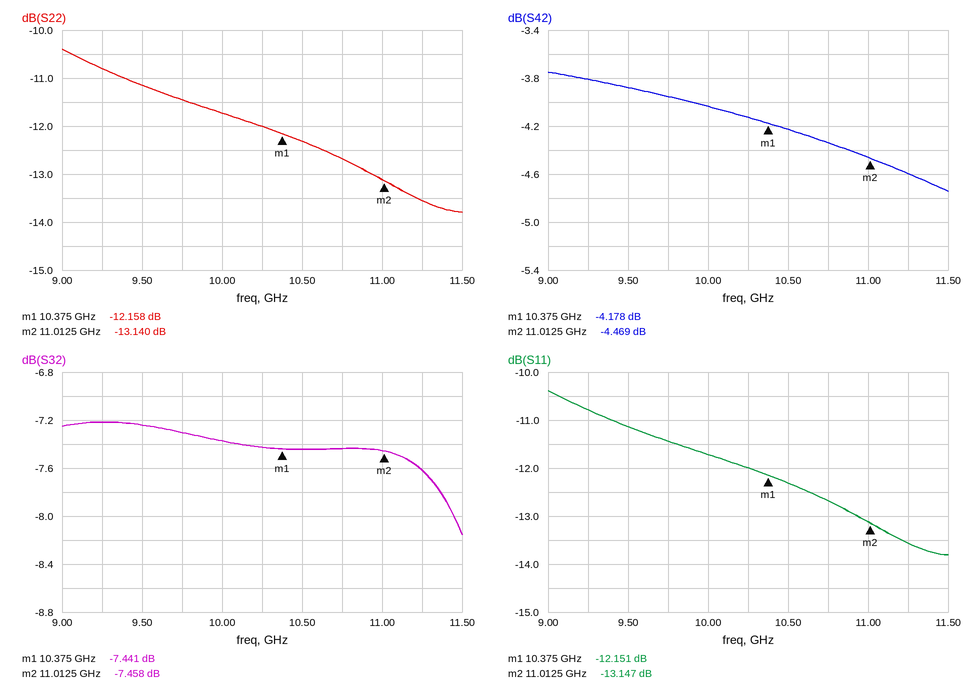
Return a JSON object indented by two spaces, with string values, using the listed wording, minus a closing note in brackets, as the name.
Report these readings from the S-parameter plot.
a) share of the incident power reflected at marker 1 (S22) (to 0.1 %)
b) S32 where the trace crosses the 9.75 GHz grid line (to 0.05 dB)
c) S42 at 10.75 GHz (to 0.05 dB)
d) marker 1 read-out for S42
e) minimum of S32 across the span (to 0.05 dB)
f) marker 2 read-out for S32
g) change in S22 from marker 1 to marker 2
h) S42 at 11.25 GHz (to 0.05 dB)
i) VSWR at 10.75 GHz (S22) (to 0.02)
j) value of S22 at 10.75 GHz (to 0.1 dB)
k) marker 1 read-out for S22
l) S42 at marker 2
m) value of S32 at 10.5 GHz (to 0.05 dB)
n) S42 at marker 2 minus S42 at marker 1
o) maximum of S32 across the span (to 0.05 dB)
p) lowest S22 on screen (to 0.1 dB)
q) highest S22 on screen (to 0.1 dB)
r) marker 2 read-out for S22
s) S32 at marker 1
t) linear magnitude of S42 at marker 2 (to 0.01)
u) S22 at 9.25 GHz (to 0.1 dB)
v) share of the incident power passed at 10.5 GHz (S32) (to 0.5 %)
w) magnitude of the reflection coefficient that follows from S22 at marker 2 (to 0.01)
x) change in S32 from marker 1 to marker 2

{
  "share of the incident power reflected at marker 1 (S22)": "6.1 %",
  "S32 where the trace crosses the 9.75 GHz grid line": "-7.30 dB",
  "S42 at 10.75 GHz": "-4.35 dB",
  "marker 1 read-out for S42": "-4.178 dB",
  "minimum of S32 across the span": "-8.15 dB",
  "marker 2 read-out for S32": "-7.458 dB",
  "change in S22 from marker 1 to marker 2": "-0.982 dB",
  "S42 at 11.25 GHz": "-4.60 dB",
  "VSWR at 10.75 GHz (S22)": "1.60",
  "value of S22 at 10.75 GHz": "-12.7 dB",
  "marker 1 read-out for S22": "-12.158 dB",
  "S42 at marker 2": "-4.469 dB",
  "value of S32 at 10.5 GHz": "-7.45 dB",
  "S42 at marker 2 minus S42 at marker 1": "-0.291 dB",
  "maximum of S32 across the span": "-7.20 dB",
  "lowest S22 on screen": "-13.8 dB",
  "highest S22 on screen": "-10.4 dB",
  "marker 2 read-out for S22": "-13.140 dB",
  "S32 at marker 1": "-7.441 dB",
  "linear magnitude of S42 at marker 2": "0.60",
  "S22 at 9.25 GHz": "-10.8 dB",
  "share of the incident power passed at 10.5 GHz (S32)": "18.0 %",
  "magnitude of the reflection coefficient that follows from S22 at marker 2": "0.22",
  "change in S32 from marker 1 to marker 2": "-0.017 dB"
}
